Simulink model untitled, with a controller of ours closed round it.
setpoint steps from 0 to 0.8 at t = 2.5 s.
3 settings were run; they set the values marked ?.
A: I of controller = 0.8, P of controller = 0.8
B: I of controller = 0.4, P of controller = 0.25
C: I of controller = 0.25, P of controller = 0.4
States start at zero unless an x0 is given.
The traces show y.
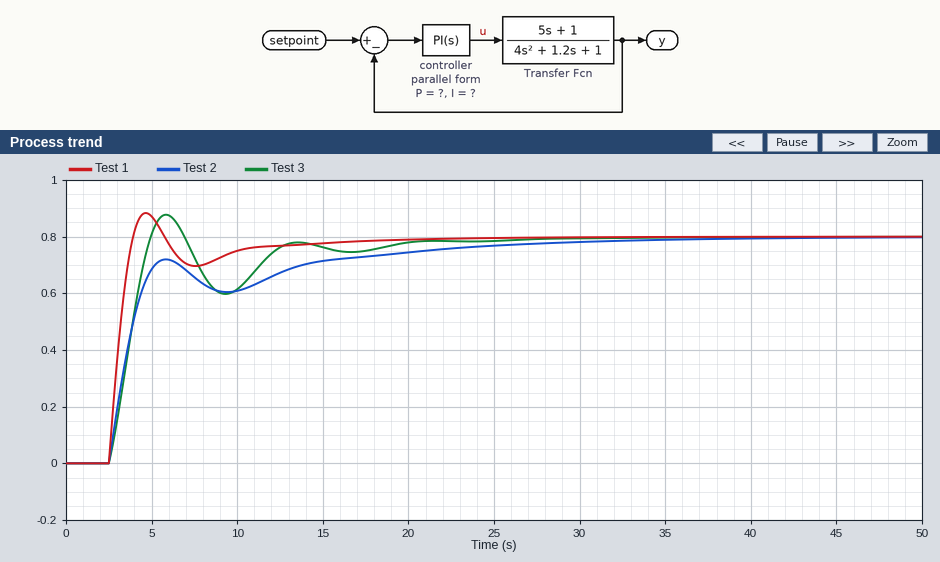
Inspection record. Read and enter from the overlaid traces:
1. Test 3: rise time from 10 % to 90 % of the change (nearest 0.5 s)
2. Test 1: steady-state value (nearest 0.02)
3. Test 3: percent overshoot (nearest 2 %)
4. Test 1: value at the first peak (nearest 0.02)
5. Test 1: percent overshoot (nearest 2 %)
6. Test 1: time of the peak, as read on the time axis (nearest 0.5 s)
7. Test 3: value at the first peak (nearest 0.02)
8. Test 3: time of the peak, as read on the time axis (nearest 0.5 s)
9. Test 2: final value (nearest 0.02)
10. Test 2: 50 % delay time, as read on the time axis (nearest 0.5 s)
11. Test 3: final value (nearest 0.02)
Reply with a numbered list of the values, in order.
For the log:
1. 2.0 s
2. 0.80
3. 10 %
4. 0.88
5. 10 %
6. 4.5 s
7. 0.88
8. 6.0 s
9. 0.80
10. 3.5 s
11. 0.80
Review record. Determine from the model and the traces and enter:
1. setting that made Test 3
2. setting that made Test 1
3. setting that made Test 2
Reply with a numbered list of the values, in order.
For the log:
1. B
2. A
3. C
